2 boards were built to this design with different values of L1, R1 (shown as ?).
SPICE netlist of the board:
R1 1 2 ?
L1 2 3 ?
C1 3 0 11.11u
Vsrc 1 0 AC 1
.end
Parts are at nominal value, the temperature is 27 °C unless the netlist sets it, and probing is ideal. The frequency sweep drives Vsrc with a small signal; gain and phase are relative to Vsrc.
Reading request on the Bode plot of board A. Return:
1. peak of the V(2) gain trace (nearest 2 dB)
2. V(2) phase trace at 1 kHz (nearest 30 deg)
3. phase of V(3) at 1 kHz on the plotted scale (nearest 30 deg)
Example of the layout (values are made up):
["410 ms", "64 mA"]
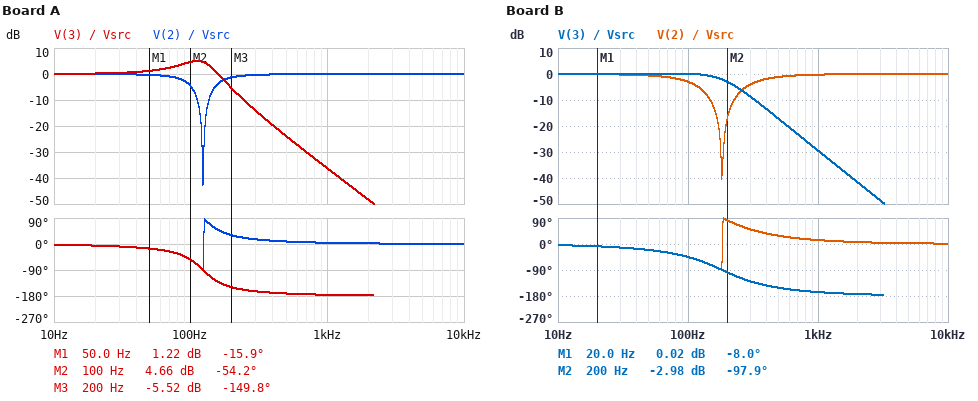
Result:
["0 dB", "0 deg", "-180 deg"]
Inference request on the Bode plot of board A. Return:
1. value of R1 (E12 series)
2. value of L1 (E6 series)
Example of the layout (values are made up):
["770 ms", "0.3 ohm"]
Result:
["68 Ω", "150 mH"]
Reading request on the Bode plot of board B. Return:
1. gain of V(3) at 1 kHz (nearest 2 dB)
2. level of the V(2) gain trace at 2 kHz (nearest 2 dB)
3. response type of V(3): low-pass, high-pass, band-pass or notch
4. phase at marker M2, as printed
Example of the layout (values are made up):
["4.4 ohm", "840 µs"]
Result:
["-30 dB", "0 dB", "low-pass", "-97.9 deg"]
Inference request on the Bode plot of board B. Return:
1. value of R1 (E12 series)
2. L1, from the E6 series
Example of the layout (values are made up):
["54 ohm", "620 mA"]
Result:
["100 Ω", "68 mH"]
